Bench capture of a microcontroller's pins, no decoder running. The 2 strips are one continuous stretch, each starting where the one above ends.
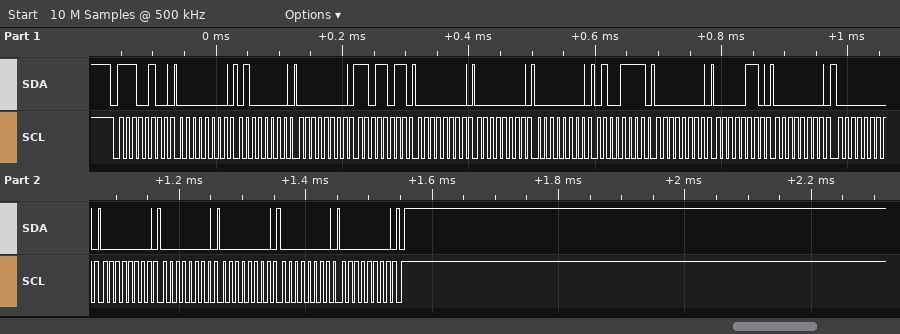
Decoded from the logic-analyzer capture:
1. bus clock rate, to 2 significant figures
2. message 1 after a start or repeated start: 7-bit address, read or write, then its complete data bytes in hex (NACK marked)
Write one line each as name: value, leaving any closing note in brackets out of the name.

bus clock rate, to 2 significant figures: 100 kHz
message 1 after a start or repeated start: 7-bit address, read or write, then its complete data bytes in hex: 0x72 write: 00 40 00 DB 00 00 00 4F 00 06 00 00 00 00 00 00 00
